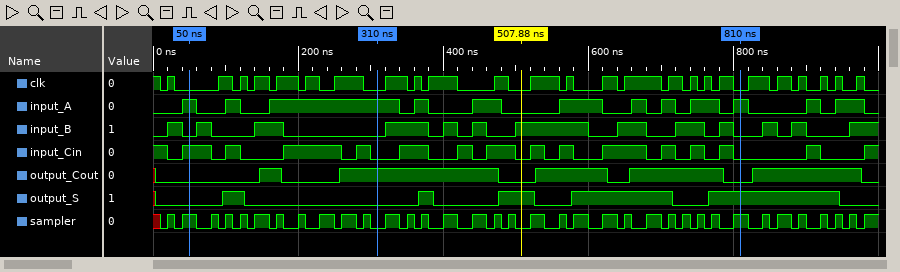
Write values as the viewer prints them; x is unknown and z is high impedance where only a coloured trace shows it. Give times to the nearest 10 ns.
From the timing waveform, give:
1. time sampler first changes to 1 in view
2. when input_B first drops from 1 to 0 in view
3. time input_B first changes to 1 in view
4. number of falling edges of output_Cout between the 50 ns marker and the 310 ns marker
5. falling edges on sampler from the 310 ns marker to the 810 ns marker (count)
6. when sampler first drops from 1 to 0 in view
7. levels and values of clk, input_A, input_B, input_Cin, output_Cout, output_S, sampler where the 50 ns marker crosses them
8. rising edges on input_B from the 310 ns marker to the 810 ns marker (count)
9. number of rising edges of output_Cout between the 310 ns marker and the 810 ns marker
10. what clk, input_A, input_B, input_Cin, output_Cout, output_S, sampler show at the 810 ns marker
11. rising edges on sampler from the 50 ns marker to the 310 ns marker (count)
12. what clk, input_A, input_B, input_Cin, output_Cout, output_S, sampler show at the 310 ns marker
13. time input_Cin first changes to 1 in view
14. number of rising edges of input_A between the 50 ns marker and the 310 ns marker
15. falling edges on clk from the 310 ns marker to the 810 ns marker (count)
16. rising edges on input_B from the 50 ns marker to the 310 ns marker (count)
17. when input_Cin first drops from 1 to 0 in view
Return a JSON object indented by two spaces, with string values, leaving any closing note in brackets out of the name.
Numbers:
{
  "time sampler first changes to 1 in view": "20 ns",
  "when input_B first drops from 1 to 0 in view": "40 ns",
  "time input_B first changes to 1 in view": "20 ns",
  "number of falling edges of output_Cout between the 50 ns marker and the 310 ns marker": "1",
  "falling edges on sampler from the 310 ns marker to the 810 ns marker": "17",
  "when sampler first drops from 1 to 0 in view": "30 ns",
  "levels and values of clk, input_A, input_B, input_Cin, output_Cout, output_S, sampler where the 50 ns marker crosses them": "clk=0, input_A=1, input_B=0, input_Cin=1, output_Cout=0, output_S=0, sampler=1",
  "rising edges on input_B from the 310 ns marker to the 810 ns marker": "7",
  "number of rising edges of output_Cout between the 310 ns marker and the 810 ns marker": "2",
  "what clk, input_A, input_B, input_Cin, output_Cout, output_S, sampler show at the 810 ns marker": "clk=0, input_A=1, input_B=0, input_Cin=0, output_Cout=0, output_S=1, sampler=1",
  "rising edges on sampler from the 50 ns marker to the 310 ns marker": "9",
  "what clk, input_A, input_B, input_Cin, output_Cout, output_S, sampler show at the 310 ns marker": "clk=0, input_A=1, input_B=0, input_Cin=0, output_Cout=1, output_S=0, sampler=0",
  "time input_Cin first changes to 1 in view": "40 ns",
  "number of rising edges of input_A between the 50 ns marker and the 310 ns marker": "2",
  "falling edges on clk from the 310 ns marker to the 810 ns marker": "12",
  "rising edges on input_B from the 50 ns marker to the 310 ns marker": "2",
  "when input_Cin first drops from 1 to 0 in view": "20 ns"
}
